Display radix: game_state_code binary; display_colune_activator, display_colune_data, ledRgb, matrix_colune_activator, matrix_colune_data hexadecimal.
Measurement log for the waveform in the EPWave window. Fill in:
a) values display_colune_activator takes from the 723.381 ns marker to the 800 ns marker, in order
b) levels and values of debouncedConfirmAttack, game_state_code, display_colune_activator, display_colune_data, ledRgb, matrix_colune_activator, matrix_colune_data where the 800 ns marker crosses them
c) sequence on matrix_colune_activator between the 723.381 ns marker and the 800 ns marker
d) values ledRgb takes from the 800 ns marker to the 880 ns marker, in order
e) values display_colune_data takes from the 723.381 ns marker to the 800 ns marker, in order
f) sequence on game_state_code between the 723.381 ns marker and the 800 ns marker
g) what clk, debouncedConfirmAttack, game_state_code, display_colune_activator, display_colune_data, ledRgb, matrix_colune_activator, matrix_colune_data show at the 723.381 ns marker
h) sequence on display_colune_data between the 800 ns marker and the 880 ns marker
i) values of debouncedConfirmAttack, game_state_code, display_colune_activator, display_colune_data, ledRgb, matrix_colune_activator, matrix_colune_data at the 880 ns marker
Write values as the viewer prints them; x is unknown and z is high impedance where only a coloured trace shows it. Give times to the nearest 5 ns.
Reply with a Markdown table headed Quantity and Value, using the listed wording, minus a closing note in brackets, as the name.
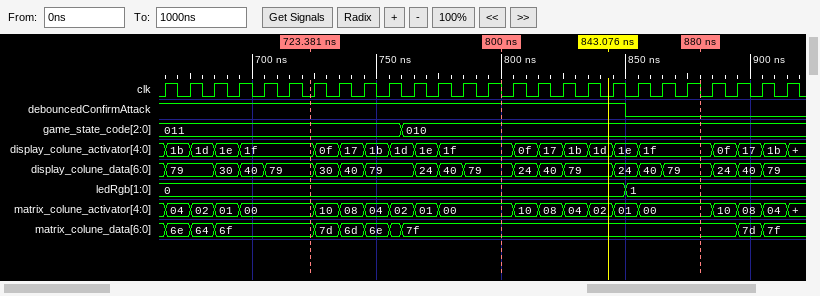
| Quantity | Value |
|---|---|
| values display_colune_activator takes from the 723.381 ns marker to the 800 ns marker, in order | 1f, 0f, 17, 1b, 1d, 1e, 1f |
| levels and values of debouncedConfirmAttack, game_state_code, display_colune_activator, display_colune_data, ledRgb, matrix_colune_activator, matrix_colune_data where the 800 ns marker crosses them | debouncedConfirmAttack=1, game_state_code=010, display_colune_activator=1f, display_colune_data=79, ledRgb=0, matrix_colune_activator=00, matrix_colune_data=7f |
| sequence on matrix_colune_activator between the 723.381 ns marker and the 800 ns marker | 00, 10, 08, 04, 02, 01, 00 |
| values ledRgb takes from the 800 ns marker to the 880 ns marker, in order | 0, 1 |
| values display_colune_data takes from the 723.381 ns marker to the 800 ns marker, in order | 79, 30, 40, 79, 24, 40, 79 |
| sequence on game_state_code between the 723.381 ns marker and the 800 ns marker | 011, 010 |
| what clk, debouncedConfirmAttack, game_state_code, display_colune_activator, display_colune_data, ledRgb, matrix_colune_activator, matrix_colune_data show at the 723.381 ns marker | clk=0, debouncedConfirmAttack=1, game_state_code=011, display_colune_activator=1f, display_colune_data=79, ledRgb=0, matrix_colune_activator=00, matrix_colune_data=6f |
| sequence on display_colune_data between the 800 ns marker and the 880 ns marker | 79, 24, 40, 79, 24, 40, 79 |
| values of debouncedConfirmAttack, game_state_code, display_colune_activator, display_colune_data, ledRgb, matrix_colune_activator, matrix_colune_data at the 880 ns marker | debouncedConfirmAttack=0, game_state_code=010, display_colune_activator=1f, display_colune_data=79, ledRgb=1, matrix_colune_activator=00, matrix_colune_data=7f |
